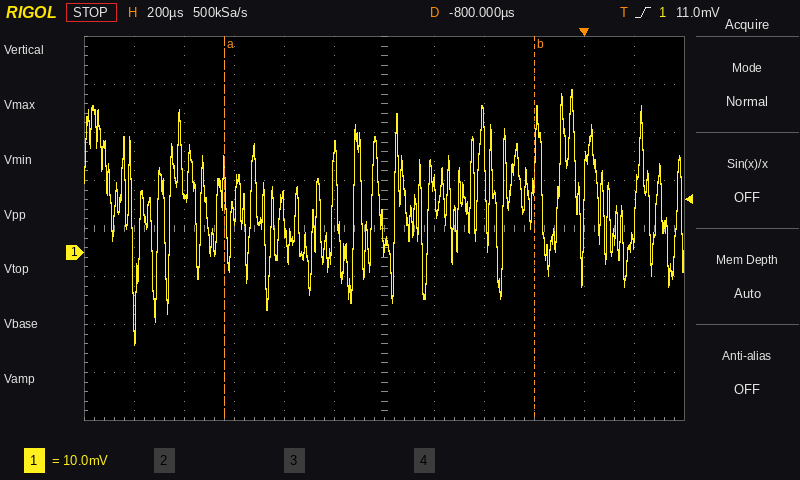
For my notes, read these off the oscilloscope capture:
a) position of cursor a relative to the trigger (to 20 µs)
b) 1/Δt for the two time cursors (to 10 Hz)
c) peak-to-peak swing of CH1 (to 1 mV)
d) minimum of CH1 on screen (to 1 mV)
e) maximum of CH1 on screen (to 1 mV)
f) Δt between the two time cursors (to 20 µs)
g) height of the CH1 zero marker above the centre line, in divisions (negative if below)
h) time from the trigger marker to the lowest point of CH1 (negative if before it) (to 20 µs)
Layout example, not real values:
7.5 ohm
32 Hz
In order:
-1.44 ms
810 Hz
53 mV
-19 mV
34 mV
1.24 ms
-0.5 div
-1.80 ms
